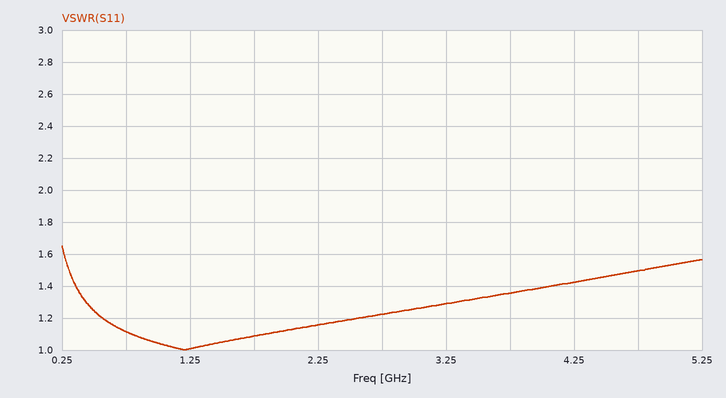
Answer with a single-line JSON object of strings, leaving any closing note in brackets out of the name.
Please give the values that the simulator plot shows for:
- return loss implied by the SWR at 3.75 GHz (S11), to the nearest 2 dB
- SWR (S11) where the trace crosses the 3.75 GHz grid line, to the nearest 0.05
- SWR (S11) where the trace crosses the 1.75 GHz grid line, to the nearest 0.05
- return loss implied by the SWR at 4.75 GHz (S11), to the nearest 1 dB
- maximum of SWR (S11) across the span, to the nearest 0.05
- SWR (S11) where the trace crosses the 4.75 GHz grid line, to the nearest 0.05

{"return loss implied by the SWR at 3.75 GHz (S11), to the nearest 2 dB": "16 dB", "SWR (S11) where the trace crosses the 3.75 GHz grid line, to the nearest 0.05": "1.35", "SWR (S11) where the trace crosses the 1.75 GHz grid line, to the nearest 0.05": "1.10", "return loss implied by the SWR at 4.75 GHz (S11), to the nearest 1 dB": "14 dB", "maximum of SWR (S11) across the span, to the nearest 0.05": "1.65", "SWR (S11) where the trace crosses the 4.75 GHz grid line, to the nearest 0.05": "1.50"}
